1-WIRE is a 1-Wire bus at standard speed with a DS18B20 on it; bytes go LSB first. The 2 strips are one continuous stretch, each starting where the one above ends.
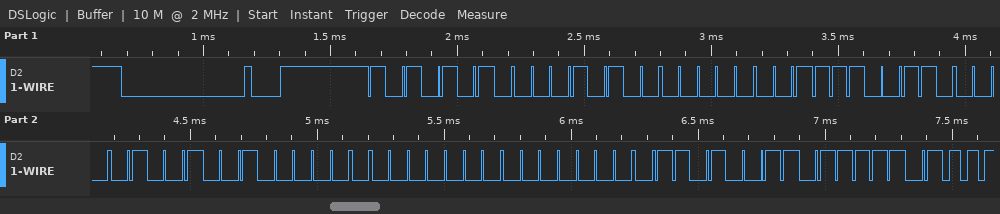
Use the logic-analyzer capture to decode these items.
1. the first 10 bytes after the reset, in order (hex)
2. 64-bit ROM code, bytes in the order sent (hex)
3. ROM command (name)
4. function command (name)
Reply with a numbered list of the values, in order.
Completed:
1. 55 28 80 67 90 04 00 00 CB BE
2. 28 80 67 90 04 00 00 CB
3. Match ROM
4. Read Scratchpad
